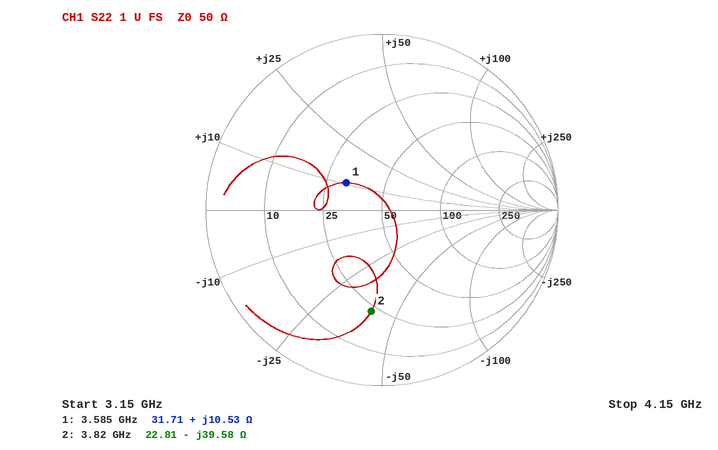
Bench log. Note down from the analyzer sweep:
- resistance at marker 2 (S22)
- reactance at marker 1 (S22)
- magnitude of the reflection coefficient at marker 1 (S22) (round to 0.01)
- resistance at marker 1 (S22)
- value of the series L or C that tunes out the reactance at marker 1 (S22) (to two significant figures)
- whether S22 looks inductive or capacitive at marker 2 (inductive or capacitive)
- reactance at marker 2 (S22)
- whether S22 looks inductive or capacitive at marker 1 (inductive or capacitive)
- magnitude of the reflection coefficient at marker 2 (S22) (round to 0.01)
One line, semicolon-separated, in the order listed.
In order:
22.81 Ω; +10.53 Ω; 0.26; 31.71 Ω; 4.2 pF; capacitive; -39.58 Ω; inductive; 0.58
